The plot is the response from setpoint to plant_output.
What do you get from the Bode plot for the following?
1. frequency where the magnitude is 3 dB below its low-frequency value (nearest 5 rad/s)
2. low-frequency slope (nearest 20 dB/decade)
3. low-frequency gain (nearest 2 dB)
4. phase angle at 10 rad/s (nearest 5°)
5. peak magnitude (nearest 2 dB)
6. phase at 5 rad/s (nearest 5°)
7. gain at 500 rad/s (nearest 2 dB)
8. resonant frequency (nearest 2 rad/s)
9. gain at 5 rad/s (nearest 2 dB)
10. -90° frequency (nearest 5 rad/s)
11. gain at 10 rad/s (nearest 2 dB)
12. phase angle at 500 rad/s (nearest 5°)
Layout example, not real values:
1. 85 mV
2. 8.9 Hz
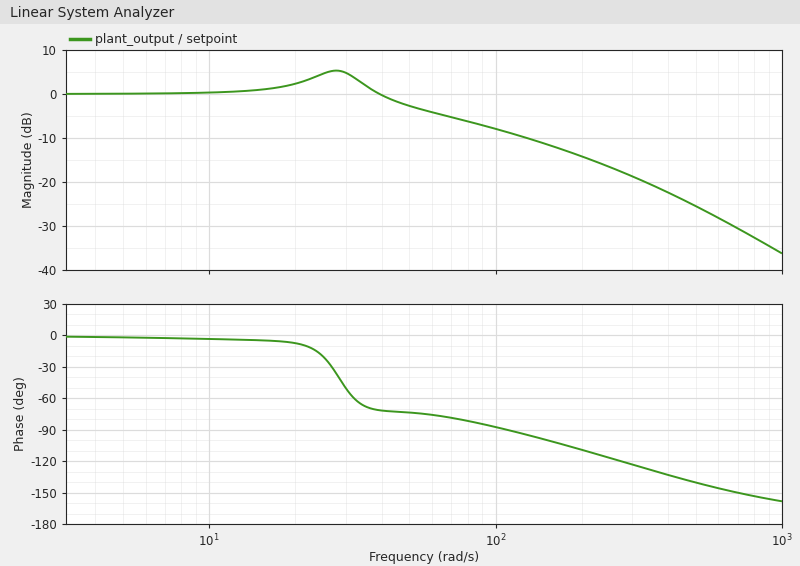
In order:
1. 50 rad/s
2. 0 dB/decade
3. 0 dB
4. -5°
5. 6 dB
6. 0°
7. -26 dB
8. 28 rad/s
9. 0 dB
10. 110 rad/s
11. 0 dB
12. -140°
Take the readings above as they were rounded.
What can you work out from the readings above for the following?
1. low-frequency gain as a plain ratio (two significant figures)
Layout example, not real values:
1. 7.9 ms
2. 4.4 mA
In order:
1. 1.0
